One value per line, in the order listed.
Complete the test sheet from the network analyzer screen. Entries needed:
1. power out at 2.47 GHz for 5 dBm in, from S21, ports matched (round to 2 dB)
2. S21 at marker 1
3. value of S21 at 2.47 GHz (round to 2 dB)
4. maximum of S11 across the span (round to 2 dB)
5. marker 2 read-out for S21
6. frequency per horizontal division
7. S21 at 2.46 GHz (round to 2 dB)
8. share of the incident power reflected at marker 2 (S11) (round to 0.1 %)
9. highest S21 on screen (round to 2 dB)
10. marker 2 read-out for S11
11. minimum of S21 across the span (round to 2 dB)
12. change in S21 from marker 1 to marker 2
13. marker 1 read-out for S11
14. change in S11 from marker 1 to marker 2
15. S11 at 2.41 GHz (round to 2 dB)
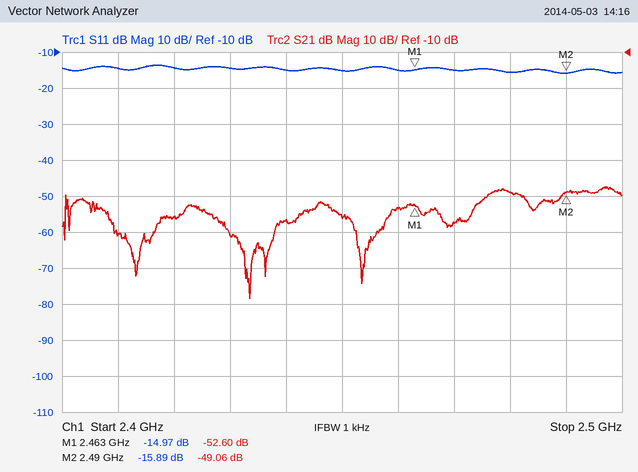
-52 dBm
-52.60 dB
-58 dB
-14 dB
-49.06 dB
10 MHz
-54 dB
2.6 %
-48 dB
-15.89 dB
-78 dB
3.54 dB
-14.97 dB
-0.92 dB
-14 dB
